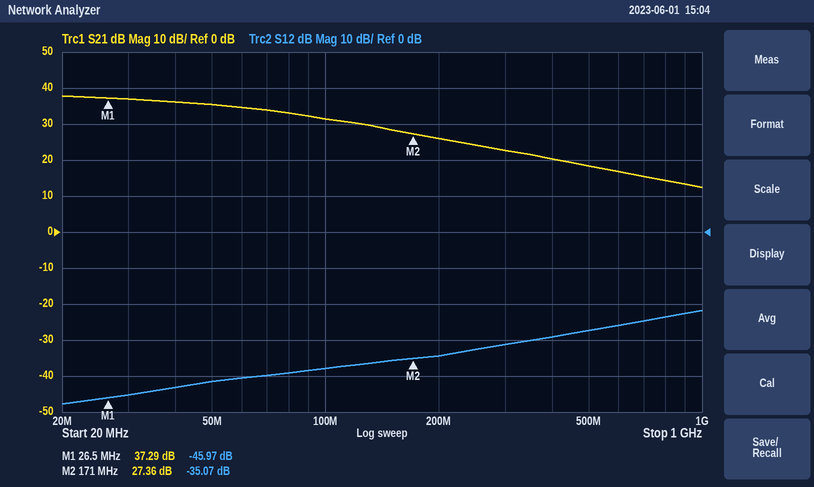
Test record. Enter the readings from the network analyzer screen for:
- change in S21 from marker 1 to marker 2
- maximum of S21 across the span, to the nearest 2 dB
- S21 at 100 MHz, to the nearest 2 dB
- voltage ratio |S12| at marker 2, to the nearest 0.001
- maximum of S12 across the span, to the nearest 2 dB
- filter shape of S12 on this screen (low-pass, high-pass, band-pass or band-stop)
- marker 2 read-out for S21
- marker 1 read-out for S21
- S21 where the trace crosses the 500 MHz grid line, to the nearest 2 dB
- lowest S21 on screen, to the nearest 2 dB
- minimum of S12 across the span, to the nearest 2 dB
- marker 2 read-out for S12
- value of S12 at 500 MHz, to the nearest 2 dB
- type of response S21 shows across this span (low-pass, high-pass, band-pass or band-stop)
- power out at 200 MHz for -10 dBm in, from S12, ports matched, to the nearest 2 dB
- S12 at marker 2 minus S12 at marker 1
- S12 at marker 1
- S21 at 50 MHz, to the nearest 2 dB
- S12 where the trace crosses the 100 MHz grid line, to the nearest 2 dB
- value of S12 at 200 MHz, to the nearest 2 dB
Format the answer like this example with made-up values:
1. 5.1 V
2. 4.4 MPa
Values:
1. -9.93 dB
2. 38 dB
3. 32 dB
4. 0.018
5. -22 dB
6. high-pass
7. 27.36 dB
8. 37.29 dB
9. 18 dB
10. 12 dB
11. -48 dB
12. -35.07 dB
13. -28 dB
14. low-pass
15. -44 dBm
16. 10.90 dB
17. -45.97 dB
18. 36 dB
19. -38 dB
20. -34 dB
